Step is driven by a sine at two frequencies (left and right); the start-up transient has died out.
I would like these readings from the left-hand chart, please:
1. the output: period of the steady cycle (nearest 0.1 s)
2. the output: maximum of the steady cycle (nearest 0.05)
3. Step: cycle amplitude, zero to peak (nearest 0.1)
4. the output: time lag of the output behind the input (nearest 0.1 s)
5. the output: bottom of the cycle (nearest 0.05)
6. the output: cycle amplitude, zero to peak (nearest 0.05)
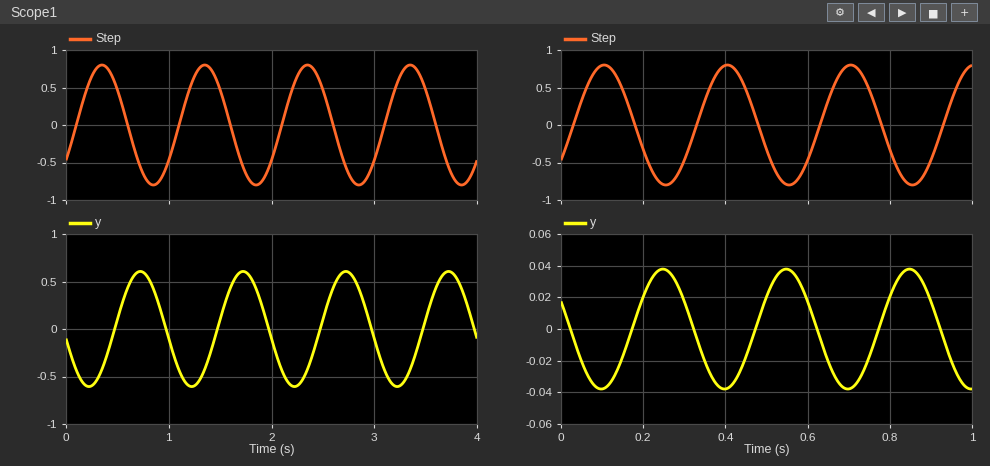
1.0 s
0.60
0.8
0.4 s
-0.60
0.60
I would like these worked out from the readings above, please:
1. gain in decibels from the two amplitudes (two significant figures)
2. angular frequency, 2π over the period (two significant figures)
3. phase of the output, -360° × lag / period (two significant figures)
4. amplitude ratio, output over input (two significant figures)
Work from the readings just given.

-2.5 dB
6.3 rad/s
-140°
0.75
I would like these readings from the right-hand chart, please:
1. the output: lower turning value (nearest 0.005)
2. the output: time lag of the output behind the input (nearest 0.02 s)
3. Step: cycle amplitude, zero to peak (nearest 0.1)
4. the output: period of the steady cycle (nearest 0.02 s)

-0.040
0.14 s
0.8
0.30 s
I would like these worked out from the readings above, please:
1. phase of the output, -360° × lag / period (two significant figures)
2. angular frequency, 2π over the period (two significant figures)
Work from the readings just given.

-170°
21 rad/s
